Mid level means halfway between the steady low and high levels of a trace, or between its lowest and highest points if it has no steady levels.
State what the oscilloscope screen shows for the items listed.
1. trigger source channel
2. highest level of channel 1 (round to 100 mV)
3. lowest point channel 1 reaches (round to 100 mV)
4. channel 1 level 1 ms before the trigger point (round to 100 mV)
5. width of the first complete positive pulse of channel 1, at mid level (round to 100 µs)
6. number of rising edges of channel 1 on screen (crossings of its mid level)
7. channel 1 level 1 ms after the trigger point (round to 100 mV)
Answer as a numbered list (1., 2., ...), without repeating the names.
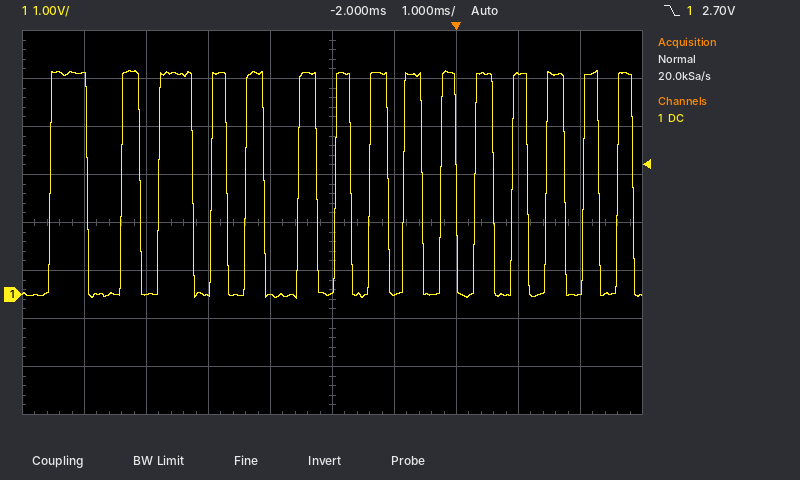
1. channel 1
2. 4.7 V
3. -100 mV
4. 0.0 V
5. 600 µs
6. 15
7. 4.6 V
